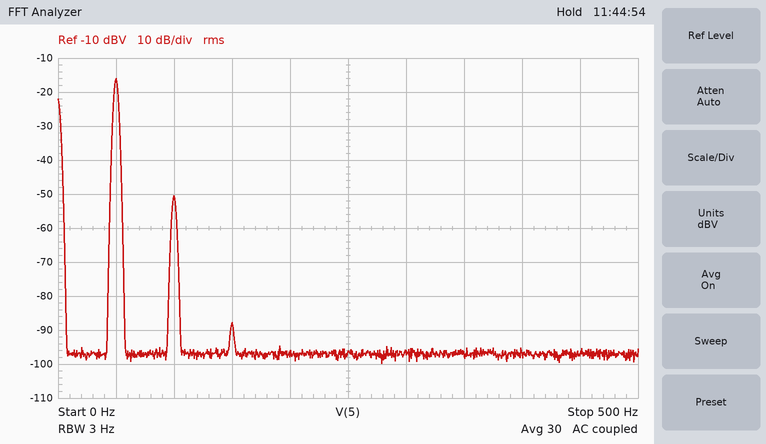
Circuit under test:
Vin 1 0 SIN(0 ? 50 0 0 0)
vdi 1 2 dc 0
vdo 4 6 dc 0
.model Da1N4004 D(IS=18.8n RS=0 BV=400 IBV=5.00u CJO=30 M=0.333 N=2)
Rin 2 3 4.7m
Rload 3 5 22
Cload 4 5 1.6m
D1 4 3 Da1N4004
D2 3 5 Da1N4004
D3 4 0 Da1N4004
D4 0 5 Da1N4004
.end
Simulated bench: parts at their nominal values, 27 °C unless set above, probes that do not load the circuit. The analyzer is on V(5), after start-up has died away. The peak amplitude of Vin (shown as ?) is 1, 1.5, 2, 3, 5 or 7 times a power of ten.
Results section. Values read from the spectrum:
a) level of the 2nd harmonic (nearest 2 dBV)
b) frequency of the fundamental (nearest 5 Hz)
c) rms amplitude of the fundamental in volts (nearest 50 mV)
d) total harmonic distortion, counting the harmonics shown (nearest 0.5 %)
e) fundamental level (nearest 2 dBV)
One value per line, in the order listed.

-50 dBV
50 Hz
150 mV
2.0 %
-16 dBV
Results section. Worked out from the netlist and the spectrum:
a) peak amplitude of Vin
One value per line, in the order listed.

20 V
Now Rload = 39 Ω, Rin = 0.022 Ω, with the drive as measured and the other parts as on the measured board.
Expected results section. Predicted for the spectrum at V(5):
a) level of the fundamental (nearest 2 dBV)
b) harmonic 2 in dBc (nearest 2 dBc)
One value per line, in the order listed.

-30 dBV
-48 dBc
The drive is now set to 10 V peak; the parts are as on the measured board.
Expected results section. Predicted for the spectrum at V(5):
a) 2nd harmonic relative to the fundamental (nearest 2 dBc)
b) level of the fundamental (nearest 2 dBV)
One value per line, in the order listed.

-40 dBc
-22 dBV
